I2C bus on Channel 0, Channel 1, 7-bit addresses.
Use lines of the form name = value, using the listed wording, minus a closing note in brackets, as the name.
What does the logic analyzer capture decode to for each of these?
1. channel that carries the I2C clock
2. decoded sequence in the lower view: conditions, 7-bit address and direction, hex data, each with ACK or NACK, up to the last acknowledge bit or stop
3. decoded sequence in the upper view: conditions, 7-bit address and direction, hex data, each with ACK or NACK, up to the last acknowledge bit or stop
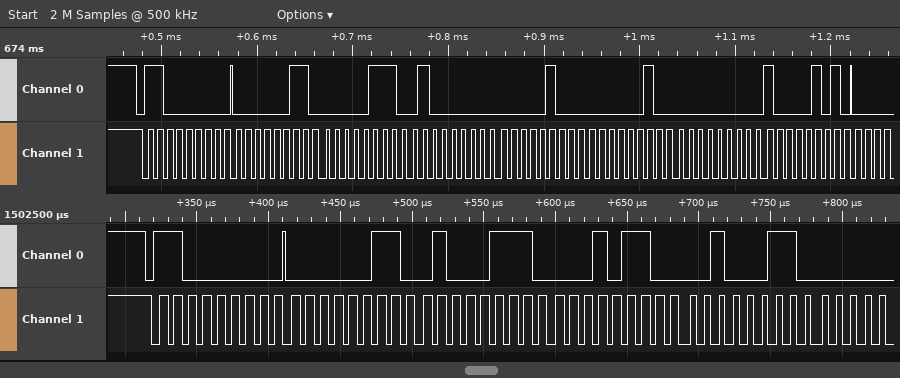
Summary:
channel that carries the I2C clock = Channel 1
decoded sequence in the lower view: conditions, 7-bit address and direction, hex data, each with ACK or NACK, up to the last acknowledge bit or stop = start, address 60 write ACK, 03 ACK, 47 ACK, 16 ACK, 23 ACK
decoded sequence in the upper view: conditions, 7-bit address and direction, hex data, each with ACK or NACK, up to the last acknowledge bit or stop = start, address 60 write ACK, 03 ACK, 07 ACK, 40 ACK, 04 ACK, 02 ACK, 00 ACK, 85 ACK
